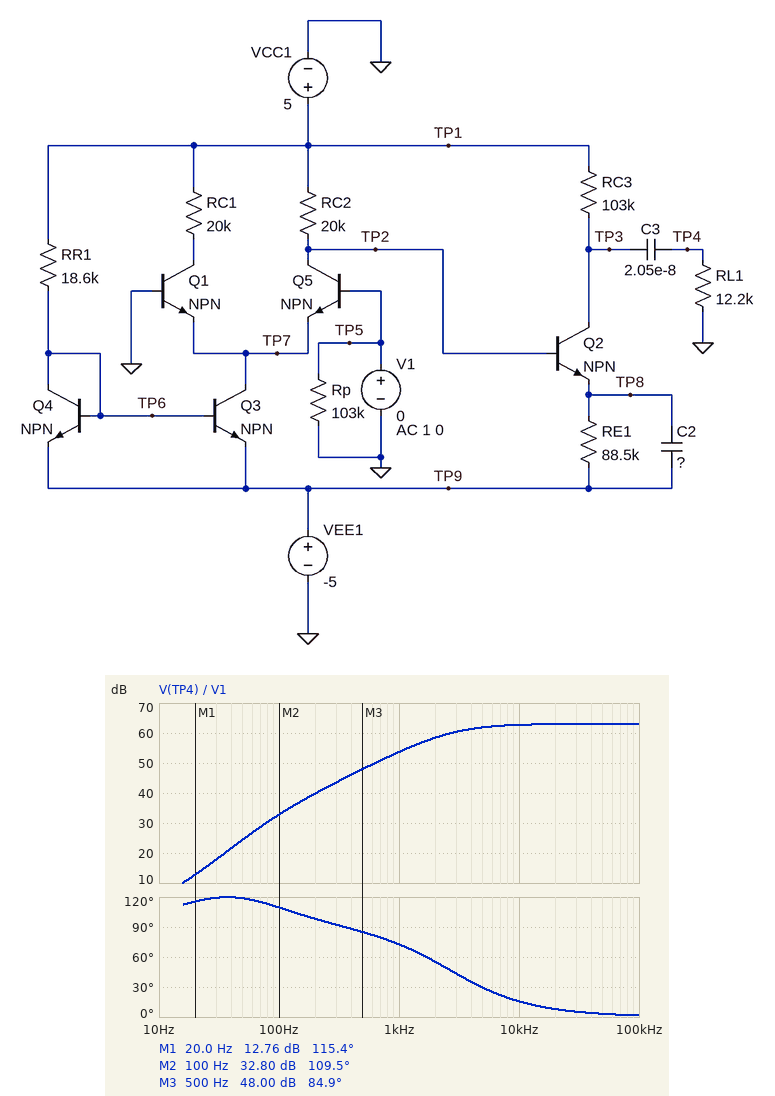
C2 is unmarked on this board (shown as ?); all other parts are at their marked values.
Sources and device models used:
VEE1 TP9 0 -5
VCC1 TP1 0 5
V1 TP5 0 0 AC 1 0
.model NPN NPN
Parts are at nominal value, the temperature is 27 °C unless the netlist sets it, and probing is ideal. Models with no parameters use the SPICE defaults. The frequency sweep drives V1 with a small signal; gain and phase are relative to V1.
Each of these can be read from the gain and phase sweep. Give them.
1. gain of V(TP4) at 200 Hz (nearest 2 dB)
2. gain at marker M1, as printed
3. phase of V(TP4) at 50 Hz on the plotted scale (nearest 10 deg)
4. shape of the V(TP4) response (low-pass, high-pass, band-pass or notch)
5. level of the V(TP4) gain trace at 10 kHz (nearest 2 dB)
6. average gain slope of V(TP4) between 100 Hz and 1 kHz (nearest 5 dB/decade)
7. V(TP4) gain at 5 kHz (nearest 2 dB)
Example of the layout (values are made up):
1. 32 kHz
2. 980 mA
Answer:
1. 40 dB
2. 12.76 dB
3. 120 deg
4. high-pass
5. 62 dB
6. 20 dB/decade
7. 62 dB
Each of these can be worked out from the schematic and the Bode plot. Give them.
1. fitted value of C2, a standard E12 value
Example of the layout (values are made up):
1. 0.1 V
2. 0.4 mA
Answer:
1. 82 nF
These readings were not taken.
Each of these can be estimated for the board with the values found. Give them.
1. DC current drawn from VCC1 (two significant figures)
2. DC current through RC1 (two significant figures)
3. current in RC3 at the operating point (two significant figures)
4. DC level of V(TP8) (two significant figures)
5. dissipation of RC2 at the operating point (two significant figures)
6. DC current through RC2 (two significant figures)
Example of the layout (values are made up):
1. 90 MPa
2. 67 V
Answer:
1. 1.0 mA
2. 240 µA
3. 50 µA
4. -530 mV
5. 1.2 mW
6. 240 µA
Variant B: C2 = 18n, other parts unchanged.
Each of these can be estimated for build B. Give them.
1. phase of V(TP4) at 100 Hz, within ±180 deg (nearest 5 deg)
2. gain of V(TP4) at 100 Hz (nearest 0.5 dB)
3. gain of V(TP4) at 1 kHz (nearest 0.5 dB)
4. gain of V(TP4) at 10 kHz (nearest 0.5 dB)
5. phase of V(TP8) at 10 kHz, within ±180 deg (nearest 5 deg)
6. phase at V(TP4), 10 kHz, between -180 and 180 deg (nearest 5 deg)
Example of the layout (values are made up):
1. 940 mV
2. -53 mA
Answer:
1. 80 deg
2. 22.5 dB
3. 41.0 dB
4. 59.0 dB
5. 140 deg
6. 50 deg
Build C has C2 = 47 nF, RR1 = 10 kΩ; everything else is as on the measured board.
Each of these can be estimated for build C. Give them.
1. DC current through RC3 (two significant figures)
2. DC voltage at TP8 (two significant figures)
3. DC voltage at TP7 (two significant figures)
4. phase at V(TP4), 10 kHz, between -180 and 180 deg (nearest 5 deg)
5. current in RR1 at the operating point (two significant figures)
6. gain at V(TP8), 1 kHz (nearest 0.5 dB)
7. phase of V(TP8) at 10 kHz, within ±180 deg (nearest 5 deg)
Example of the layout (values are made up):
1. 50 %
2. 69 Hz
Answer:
1. 40 µA
2. -1.4 V
3. -760 mV
4. -150 deg
5. 920 µA
6. -26.0 dB
7. -60 deg
